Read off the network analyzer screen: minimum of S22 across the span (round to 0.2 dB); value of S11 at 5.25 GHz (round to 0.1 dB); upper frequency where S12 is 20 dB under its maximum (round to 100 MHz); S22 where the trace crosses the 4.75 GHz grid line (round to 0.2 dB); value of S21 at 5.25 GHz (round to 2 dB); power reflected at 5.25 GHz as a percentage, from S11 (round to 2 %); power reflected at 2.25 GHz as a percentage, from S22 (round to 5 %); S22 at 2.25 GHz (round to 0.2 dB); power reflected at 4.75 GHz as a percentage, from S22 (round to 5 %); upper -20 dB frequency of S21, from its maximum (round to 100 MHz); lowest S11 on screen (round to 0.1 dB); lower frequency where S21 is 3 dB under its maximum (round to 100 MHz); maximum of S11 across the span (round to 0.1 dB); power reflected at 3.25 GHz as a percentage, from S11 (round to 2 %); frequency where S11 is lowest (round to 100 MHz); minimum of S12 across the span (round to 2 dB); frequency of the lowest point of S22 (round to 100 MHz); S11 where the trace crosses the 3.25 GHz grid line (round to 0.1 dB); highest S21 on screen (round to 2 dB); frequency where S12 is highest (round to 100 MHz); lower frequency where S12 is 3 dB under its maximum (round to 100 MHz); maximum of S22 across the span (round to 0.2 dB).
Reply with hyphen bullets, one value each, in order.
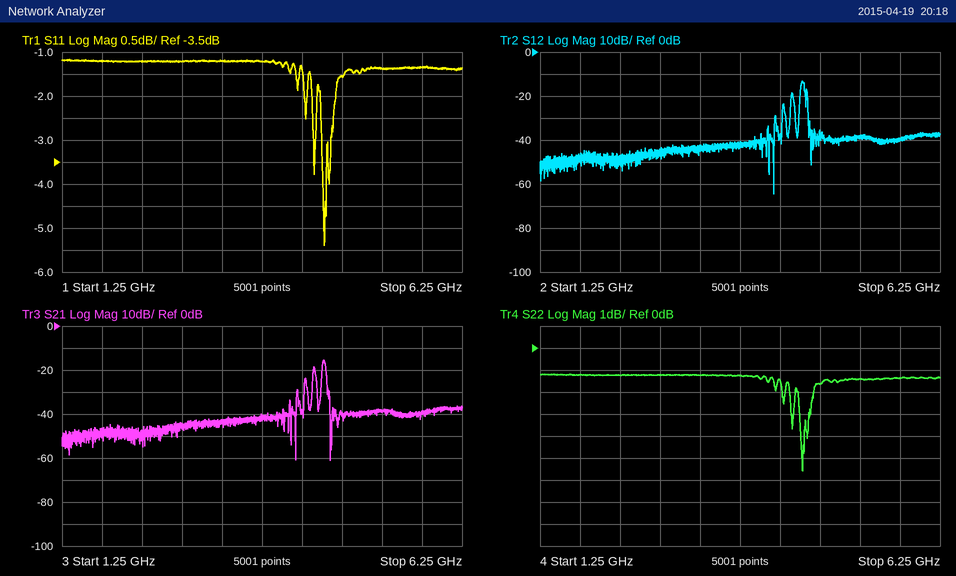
- -5.6 dB
- -1.4 dB
- 4.6 GHz
- -1.6 dB
- -38 dB
- 72 %
- 75 %
- -1.2 dB
- 70 %
- 4.6 GHz
- -5.4 dB
- 4.5 GHz
- -1.2 dB
- 76 %
- 4.5 GHz
- -64 dB
- 4.5 GHz
- -1.2 dB
- -16 dB
- 4.5 GHz
- 4.5 GHz
- -1.2 dB
